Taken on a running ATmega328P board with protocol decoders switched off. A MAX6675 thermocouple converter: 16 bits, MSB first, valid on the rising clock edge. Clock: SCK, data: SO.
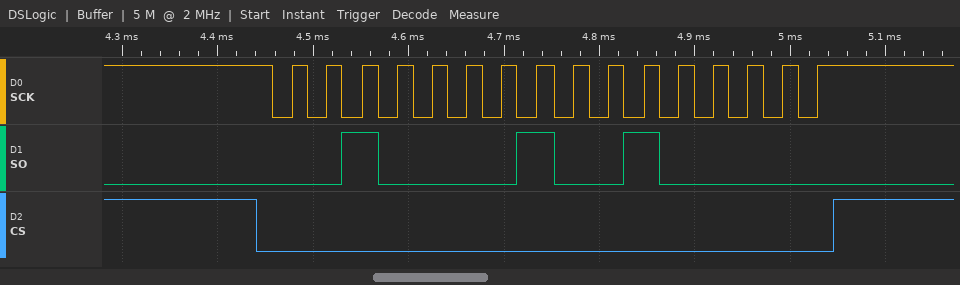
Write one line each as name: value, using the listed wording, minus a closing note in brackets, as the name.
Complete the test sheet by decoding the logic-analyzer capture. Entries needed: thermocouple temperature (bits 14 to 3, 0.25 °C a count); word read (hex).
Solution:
thermocouple temperature: 265.00 °C
word read: 0x2120
